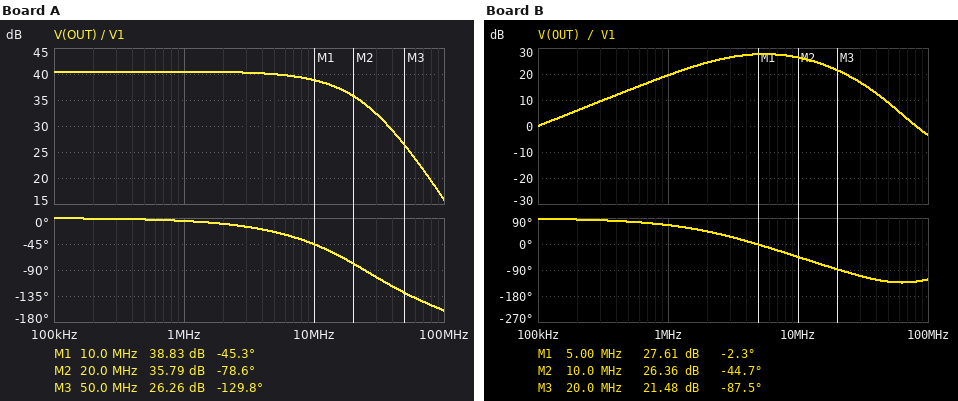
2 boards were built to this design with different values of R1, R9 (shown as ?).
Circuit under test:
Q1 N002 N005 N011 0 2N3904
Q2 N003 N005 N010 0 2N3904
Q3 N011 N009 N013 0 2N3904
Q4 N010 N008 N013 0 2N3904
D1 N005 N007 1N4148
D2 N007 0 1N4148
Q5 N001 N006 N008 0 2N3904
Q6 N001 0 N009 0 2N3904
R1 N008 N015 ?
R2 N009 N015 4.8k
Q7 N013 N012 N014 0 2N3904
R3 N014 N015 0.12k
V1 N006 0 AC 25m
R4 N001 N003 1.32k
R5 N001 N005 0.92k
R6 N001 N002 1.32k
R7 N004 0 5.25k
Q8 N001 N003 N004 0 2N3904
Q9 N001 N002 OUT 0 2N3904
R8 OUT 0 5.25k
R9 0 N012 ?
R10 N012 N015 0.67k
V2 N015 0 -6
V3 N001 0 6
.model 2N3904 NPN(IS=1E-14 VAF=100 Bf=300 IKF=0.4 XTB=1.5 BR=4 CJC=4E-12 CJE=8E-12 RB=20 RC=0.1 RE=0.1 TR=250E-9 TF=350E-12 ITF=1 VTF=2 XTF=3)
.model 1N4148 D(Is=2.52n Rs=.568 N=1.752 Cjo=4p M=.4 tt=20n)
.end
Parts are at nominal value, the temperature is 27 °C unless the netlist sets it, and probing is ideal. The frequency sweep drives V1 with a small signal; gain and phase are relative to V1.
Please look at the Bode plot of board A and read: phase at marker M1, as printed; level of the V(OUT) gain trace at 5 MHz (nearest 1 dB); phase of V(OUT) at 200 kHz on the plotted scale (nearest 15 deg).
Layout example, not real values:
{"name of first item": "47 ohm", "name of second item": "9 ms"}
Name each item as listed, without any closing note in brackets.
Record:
{"phase at marker M1, as printed": "-45.3 deg", "level of the V(OUT) gain trace at 5 MHz": "40 dB", "phase of V(OUT) at 200 kHz on the plotted scale": "0 deg"}
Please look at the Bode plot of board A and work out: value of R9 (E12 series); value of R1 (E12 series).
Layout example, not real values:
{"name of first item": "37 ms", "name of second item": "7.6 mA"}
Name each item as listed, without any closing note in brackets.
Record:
{"value of R9": "1.2 kΩ", "value of R1": "15 kΩ"}
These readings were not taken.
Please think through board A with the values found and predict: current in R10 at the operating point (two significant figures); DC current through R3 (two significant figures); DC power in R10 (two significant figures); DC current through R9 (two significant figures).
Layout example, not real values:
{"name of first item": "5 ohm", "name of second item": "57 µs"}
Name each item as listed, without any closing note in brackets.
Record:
{"current in R10 at the operating point": "3.2 mA", "DC current through R3": "12 mA", "DC power in R10": "6.8 mW", "DC current through R9": "3.2 mA"}
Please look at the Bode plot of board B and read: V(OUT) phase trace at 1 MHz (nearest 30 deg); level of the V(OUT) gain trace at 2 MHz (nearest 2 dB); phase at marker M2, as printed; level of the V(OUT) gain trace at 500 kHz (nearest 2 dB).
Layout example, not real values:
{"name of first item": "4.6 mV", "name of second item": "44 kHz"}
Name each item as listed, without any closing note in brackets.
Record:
{"V(OUT) phase trace at 1 MHz": "60 deg", "level of the V(OUT) gain trace at 2 MHz": "24 dB", "phase at marker M2, as printed": "-44.7 deg", "level of the V(OUT) gain trace at 500 kHz": "14 dB"}
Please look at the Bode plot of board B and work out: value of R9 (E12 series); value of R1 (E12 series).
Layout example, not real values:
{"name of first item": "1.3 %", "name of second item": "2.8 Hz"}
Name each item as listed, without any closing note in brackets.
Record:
{"value of R9": "1 kΩ", "value of R1": "1.8 kΩ"}
